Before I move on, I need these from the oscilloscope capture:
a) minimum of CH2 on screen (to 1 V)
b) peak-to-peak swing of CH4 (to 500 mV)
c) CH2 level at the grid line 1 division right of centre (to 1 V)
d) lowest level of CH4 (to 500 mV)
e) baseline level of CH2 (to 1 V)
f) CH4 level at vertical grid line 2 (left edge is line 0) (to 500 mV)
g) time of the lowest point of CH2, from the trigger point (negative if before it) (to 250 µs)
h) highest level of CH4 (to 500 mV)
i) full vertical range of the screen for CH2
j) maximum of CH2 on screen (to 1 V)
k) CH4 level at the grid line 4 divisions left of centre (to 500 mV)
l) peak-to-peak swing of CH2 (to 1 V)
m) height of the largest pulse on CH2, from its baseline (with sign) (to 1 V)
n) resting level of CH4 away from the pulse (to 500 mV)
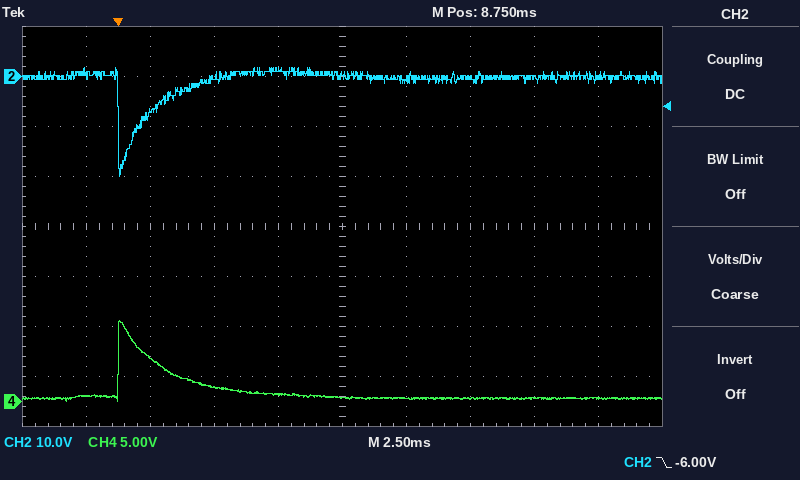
-20 V
8.0 V
-1 V
0.0 V
0 V
4.5 V
0.00 ms
8.0 V
80 V
2 V
500 mV
22 V
-20 V
500 mV
